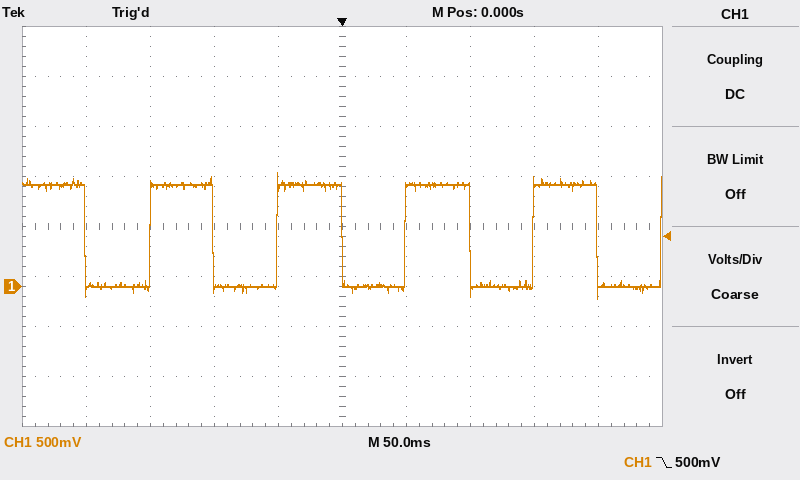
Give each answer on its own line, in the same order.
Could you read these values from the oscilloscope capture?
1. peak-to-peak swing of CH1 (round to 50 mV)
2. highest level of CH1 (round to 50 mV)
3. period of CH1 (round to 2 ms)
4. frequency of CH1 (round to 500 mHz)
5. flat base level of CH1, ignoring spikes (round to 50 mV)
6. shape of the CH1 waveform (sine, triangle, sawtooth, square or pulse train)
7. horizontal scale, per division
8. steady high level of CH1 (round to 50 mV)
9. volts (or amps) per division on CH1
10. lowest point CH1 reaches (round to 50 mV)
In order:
1.25 V
1.15 V
100 ms
10.0 Hz
0 mV
square
50 ms
1.00 V
500 mV
-100 mV
